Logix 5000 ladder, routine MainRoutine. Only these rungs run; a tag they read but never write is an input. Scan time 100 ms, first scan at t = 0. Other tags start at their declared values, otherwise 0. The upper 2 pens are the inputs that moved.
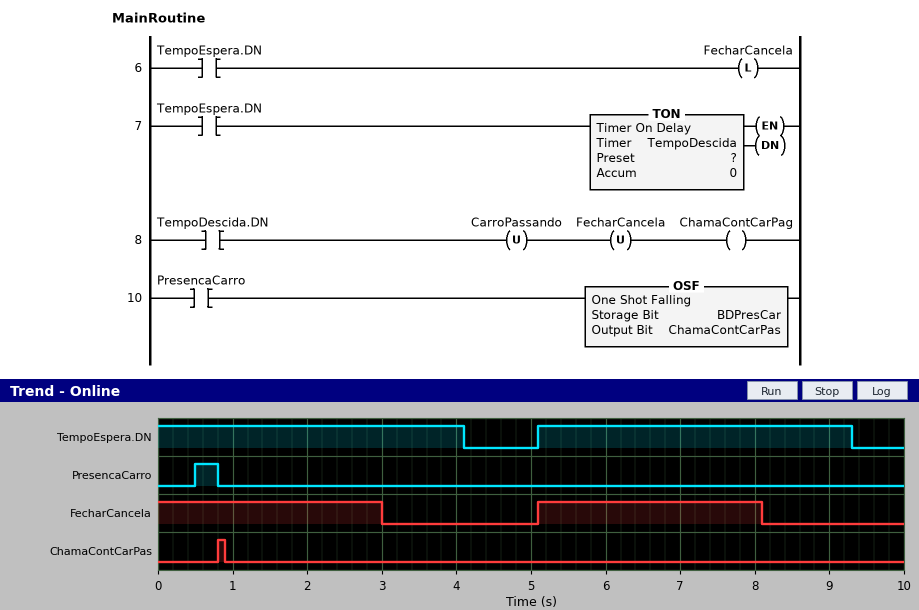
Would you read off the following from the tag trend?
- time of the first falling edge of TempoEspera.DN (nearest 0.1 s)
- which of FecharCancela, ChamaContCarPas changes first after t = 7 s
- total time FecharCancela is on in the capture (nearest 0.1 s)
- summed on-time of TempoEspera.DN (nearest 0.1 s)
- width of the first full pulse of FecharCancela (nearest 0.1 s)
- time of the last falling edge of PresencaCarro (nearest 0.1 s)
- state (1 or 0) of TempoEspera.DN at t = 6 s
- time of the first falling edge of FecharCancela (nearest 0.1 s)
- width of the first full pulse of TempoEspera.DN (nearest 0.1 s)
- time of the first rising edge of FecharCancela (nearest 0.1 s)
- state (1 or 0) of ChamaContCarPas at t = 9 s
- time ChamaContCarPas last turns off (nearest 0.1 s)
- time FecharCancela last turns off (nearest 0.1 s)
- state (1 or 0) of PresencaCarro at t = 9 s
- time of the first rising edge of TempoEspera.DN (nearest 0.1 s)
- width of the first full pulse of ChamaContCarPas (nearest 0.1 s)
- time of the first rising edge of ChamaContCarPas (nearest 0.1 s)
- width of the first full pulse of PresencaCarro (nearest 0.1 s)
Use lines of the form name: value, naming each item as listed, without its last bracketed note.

time of the first falling edge of TempoEspera.DN: 4.1 s
which of FecharCancela, ChamaContCarPas changes first after t = 7 s: FecharCancela
total time FecharCancela is on in the capture: 6.0 s
summed on-time of TempoEspera.DN: 8.3 s
width of the first full pulse of FecharCancela: 3.0 s
time of the last falling edge of PresencaCarro: 0.8 s
state (1 or 0) of TempoEspera.DN at t = 6 s: 1
time of the first falling edge of FecharCancela: 3.0 s
width of the first full pulse of TempoEspera.DN: 4.2 s
time of the first rising edge of FecharCancela: 5.1 s
state (1 or 0) of ChamaContCarPas at t = 9 s: 0
time ChamaContCarPas last turns off: 0.9 s
time FecharCancela last turns off: 8.1 s
state (1 or 0) of PresencaCarro at t = 9 s: 0
time of the first rising edge of TempoEspera.DN: 5.1 s
width of the first full pulse of ChamaContCarPas: 0.1 s
time of the first rising edge of ChamaContCarPas: 0.8 s
width of the first full pulse of PresencaCarro: 0.3 s
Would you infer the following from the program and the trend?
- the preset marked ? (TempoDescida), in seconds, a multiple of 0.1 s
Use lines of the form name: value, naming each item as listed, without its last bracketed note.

the preset marked ? (TempoDescida), in seconds, a multiple of 0.1 s: 3.0 s
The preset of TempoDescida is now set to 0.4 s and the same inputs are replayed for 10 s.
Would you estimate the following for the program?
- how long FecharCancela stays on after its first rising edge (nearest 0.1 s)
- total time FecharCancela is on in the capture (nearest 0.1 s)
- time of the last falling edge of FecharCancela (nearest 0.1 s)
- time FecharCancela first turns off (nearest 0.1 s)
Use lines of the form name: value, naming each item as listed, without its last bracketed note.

how long FecharCancela stays on after its first rising edge: 0.4 s
total time FecharCancela is on in the capture: 0.8 s
time of the last falling edge of FecharCancela: 5.5 s
time FecharCancela first turns off: 0.4 s
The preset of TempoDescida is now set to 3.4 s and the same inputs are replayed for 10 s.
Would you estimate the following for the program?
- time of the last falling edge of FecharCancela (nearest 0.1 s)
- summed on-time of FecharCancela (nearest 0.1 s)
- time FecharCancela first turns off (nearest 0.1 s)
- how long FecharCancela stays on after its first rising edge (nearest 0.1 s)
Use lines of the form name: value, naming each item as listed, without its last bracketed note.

time of the last falling edge of FecharCancela: 8.5 s
summed on-time of FecharCancela: 6.8 s
time FecharCancela first turns off: 3.4 s
how long FecharCancela stays on after its first rising edge: 3.4 s
